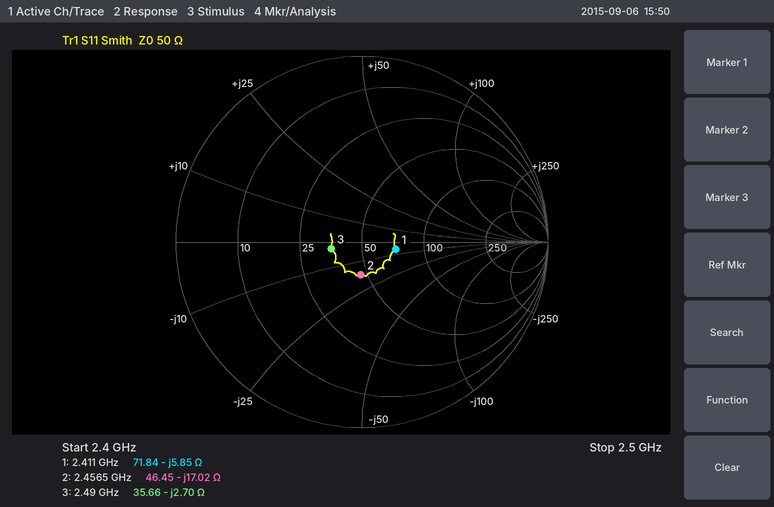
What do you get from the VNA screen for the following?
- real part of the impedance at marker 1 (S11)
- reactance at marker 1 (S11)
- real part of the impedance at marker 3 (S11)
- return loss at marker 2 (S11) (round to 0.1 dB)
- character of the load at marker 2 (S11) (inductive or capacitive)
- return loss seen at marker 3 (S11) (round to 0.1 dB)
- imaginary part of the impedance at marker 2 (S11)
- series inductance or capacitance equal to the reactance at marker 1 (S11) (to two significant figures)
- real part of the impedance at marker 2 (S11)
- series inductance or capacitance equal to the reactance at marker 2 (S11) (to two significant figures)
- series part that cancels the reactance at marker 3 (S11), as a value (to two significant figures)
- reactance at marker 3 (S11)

71.84 Ω
-5.85 Ω
35.66 Ω
15.0 dB
capacitive
15.4 dB
-17.02 Ω
11 pF
46.45 Ω
3.8 pF
170 pH
-2.70 Ω
